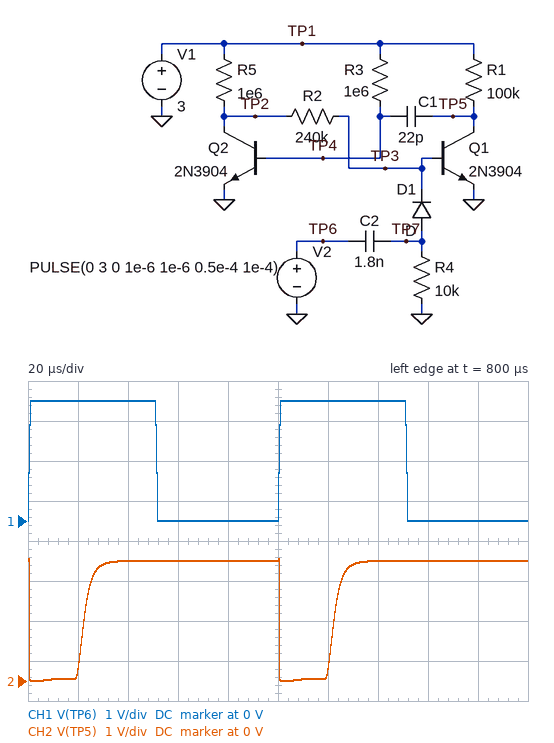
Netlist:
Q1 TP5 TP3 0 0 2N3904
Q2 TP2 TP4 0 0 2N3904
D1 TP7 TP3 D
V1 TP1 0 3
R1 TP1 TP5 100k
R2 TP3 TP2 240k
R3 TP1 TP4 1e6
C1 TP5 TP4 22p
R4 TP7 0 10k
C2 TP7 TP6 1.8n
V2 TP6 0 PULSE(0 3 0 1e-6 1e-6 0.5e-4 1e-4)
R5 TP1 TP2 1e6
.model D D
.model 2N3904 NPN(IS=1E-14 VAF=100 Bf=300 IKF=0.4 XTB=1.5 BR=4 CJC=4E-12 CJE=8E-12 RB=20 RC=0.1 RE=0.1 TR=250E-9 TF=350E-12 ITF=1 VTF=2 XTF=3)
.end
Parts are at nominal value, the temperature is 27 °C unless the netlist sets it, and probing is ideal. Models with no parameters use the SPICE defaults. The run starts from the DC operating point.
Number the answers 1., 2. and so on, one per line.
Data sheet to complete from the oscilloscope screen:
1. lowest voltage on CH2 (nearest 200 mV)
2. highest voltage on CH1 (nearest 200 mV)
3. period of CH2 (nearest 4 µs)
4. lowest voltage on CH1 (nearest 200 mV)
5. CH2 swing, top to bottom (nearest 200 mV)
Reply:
1. 0 V
2. 3.0 V
3. 100 µs
4. 0 V
5. 3.0 V
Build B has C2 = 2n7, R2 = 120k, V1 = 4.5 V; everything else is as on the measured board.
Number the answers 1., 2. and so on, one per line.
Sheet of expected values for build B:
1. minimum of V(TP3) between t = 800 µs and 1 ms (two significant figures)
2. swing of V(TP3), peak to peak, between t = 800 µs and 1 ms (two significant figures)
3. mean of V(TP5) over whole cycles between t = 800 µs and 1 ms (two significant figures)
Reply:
1. 11 mV
2. 870 mV
3. 3.6 V
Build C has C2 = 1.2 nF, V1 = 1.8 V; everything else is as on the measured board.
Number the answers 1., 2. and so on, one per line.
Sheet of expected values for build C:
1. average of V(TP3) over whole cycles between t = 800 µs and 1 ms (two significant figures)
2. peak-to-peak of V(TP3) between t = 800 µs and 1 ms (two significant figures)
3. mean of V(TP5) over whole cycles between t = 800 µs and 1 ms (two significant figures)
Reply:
1. 160 mV
2. 770 mV
3. 1.4 V
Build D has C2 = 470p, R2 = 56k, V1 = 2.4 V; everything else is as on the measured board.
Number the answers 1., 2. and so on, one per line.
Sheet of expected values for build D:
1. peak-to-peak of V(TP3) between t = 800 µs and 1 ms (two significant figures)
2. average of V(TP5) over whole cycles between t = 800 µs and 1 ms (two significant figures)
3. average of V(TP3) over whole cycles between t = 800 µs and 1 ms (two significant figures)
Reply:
1. 700 mV
2. 1.9 V
3. 130 mV
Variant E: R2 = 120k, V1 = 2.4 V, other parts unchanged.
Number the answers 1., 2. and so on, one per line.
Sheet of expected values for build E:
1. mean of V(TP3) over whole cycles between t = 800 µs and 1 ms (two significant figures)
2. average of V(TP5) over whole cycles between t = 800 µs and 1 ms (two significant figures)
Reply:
1. 140 mV
2. 1.9 V
